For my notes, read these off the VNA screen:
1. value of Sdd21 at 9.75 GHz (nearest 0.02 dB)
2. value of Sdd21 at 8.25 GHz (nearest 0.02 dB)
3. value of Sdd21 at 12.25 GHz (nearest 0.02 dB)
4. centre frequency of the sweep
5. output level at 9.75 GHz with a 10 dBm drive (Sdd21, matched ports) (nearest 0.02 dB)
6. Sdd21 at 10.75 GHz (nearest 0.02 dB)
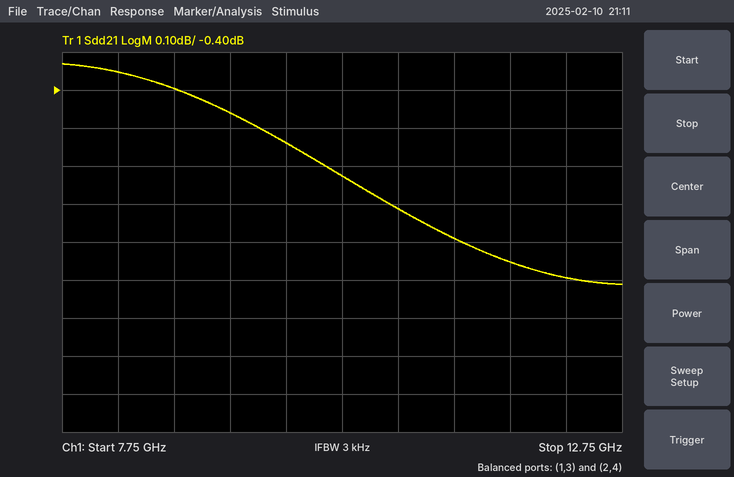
-0.54 dB
-0.36 dB
-0.90 dB
10.25 GHz
9.46 dBm
-0.72 dB
